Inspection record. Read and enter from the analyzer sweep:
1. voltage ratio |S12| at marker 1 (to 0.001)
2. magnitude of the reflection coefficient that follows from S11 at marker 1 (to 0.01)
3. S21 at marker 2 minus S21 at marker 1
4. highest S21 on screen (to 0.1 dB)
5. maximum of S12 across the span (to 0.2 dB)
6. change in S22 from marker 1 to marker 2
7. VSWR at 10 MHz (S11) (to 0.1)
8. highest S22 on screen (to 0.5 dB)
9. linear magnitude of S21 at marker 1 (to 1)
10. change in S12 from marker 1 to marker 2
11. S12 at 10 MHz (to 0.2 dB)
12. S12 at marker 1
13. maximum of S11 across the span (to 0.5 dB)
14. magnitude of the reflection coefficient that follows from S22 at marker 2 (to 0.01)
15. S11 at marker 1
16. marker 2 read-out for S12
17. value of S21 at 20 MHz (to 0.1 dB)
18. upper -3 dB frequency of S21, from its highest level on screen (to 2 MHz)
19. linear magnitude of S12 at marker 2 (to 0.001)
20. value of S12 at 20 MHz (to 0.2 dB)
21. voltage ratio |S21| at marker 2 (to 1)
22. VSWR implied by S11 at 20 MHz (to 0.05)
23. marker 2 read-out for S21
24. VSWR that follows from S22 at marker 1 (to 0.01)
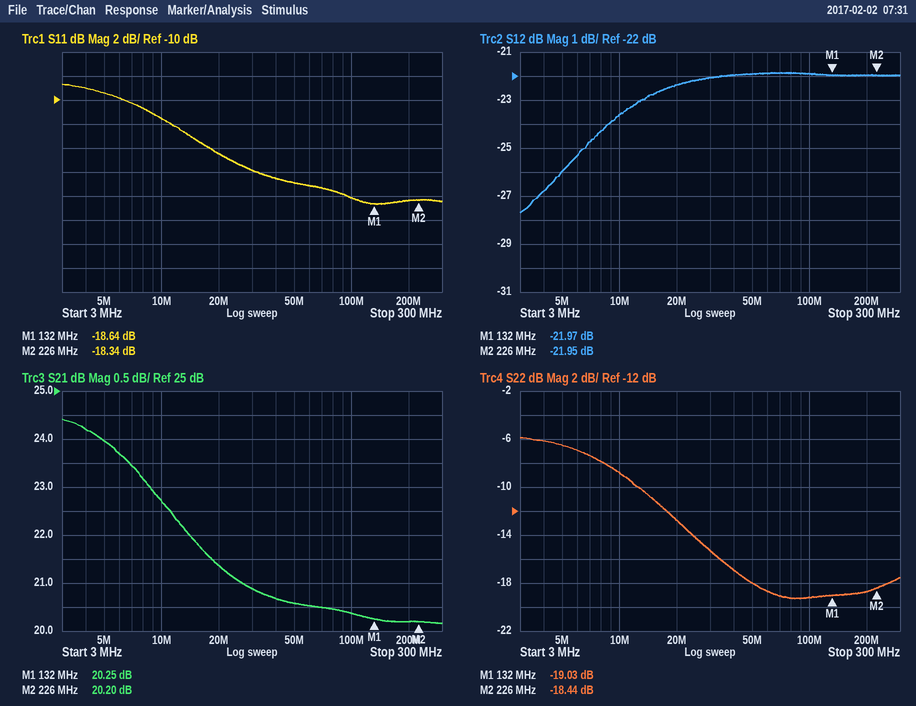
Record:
0.080
0.12
-0.05 dB
24.4 dB
-21.8 dB
0.59 dB
1.7
-6.0 dB
10
0.02 dB
-23.6 dB
-21.97 dB
-8.5 dB
0.12
-18.64 dB
-21.95 dB
21.4 dB
20 MHz
0.080
-22.4 dB
10
1.45
20.20 dB
1.25
